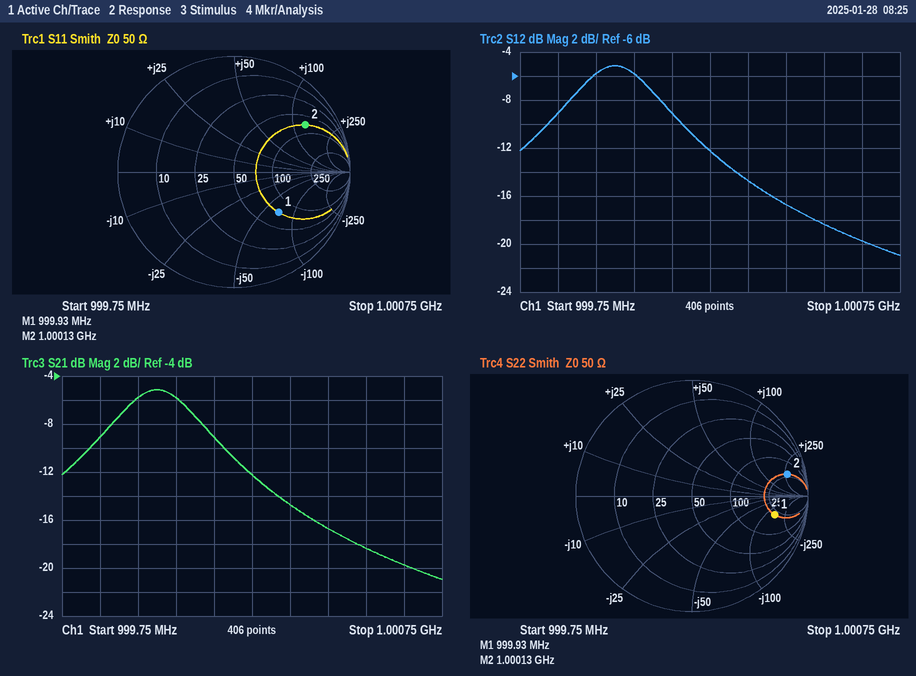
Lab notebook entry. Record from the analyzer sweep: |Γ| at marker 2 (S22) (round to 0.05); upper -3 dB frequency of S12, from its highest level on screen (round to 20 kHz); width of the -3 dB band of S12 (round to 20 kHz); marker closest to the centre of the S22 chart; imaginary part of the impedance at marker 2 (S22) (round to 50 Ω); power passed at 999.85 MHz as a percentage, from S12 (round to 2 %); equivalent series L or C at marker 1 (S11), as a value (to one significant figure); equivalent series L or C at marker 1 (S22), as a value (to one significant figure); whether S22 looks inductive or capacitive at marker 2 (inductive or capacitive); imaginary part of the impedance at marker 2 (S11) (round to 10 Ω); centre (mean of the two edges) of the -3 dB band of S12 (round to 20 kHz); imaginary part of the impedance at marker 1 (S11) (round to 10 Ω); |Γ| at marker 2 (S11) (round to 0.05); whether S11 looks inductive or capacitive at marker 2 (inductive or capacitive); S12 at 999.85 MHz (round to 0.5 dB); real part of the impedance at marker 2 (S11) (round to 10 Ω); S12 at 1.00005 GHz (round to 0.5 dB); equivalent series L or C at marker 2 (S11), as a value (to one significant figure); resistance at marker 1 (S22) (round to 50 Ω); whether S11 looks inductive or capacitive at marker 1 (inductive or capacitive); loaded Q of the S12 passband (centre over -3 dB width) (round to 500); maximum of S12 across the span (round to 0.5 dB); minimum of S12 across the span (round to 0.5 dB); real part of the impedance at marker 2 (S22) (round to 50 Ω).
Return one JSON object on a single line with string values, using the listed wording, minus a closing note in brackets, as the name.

{"|Γ| at marker 2 (S22)": "0.85", "upper -3 dB frequency of S12, from its highest level on screen": "1.00012 GHz", "width of the -3 dB band of S12": "240 kHz", "marker closest to the centre of the S22 chart": "marker 1", "imaginary part of the impedance at marker 2 (S22)": "+300 Ω", "power passed at 999.85 MHz as a percentage, from S12": "12 %", "equivalent series L or C at marker 1 (S11), as a value": "2 pF", "equivalent series L or C at marker 1 (S22), as a value": "1 pF", "whether S22 looks inductive or capacitive at marker 2": "inductive", "imaginary part of the impedance at marker 2 (S11)": "+130 Ω", "centre (mean of the two edges) of the -3 dB band of S12": "1.00000 GHz", "imaginary part of the impedance at marker 1 (S11)": "-70 Ω", "|Γ| at marker 2 (S11)": "0.75", "whether S11 looks inductive or capacitive at marker 2": "inductive", "S12 at 999.85 MHz": "-9.0 dB", "real part of the impedance at marker 2 (S11)": "70 Ω", "S12 at 1.00005 GHz": "-6.0 dB", "equivalent series L or C at marker 2 (S11), as a value": "20 nH", "resistance at marker 1 (S22)": "200 Ω", "whether S11 looks inductive or capacitive at marker 1": "capacitive", "loaded Q of the S12 passband (centre over -3 dB width)": "4000", "maximum of S12 across the span": "-5.0 dB", "minimum of S12 across the span": "-21.0 dB", "real part of the impedance at marker 2 (S22)": "200 Ω"}
